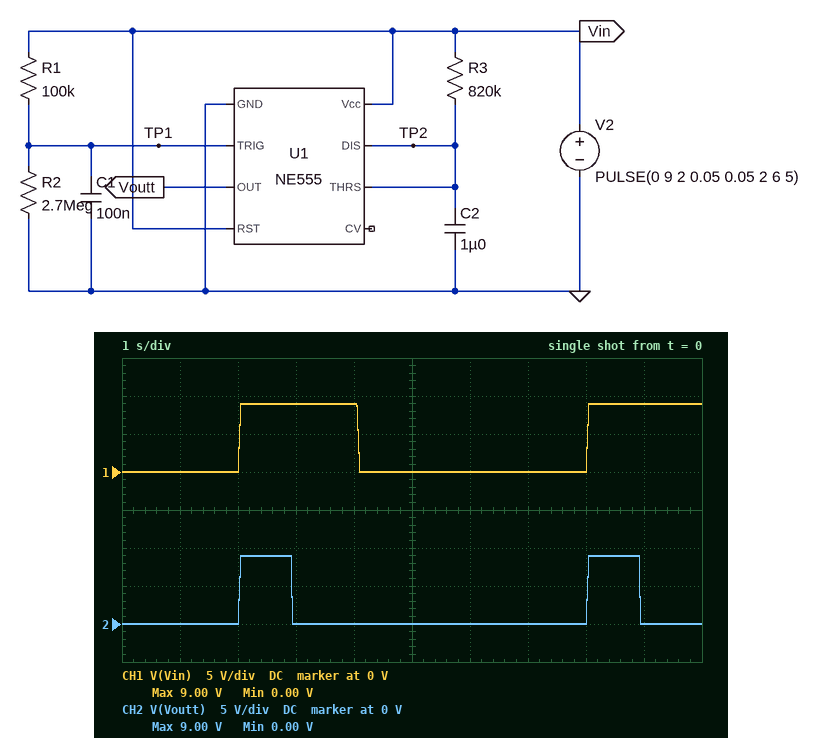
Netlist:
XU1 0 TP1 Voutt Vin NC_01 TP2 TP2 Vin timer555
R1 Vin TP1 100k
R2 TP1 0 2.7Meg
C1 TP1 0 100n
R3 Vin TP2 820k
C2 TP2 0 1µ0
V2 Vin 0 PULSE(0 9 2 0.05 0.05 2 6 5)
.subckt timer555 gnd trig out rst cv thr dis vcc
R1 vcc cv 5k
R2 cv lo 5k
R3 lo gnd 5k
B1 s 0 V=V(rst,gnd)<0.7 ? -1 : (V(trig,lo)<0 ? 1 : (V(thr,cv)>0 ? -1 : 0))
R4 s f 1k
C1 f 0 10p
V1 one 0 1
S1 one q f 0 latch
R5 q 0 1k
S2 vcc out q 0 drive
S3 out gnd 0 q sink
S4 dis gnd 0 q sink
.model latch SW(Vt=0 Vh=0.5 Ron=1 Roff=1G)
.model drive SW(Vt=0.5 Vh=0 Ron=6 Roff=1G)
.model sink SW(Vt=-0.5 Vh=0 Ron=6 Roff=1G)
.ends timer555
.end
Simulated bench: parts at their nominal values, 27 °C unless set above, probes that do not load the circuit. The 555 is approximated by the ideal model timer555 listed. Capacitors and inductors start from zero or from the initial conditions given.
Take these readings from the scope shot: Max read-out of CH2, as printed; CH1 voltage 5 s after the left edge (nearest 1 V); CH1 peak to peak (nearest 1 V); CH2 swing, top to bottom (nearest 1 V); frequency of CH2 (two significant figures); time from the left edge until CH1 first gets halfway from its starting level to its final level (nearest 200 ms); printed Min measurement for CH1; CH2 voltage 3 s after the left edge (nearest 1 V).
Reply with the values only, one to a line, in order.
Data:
9.00 V
0 V
9 V
9 V
170 mHz
2.0 s
0.00 V
0 V
